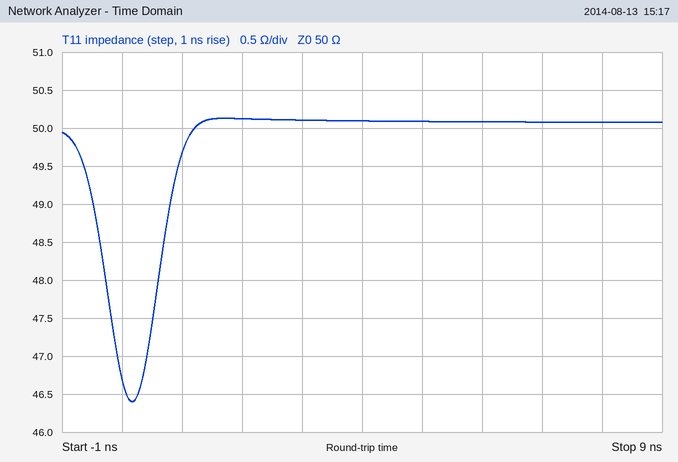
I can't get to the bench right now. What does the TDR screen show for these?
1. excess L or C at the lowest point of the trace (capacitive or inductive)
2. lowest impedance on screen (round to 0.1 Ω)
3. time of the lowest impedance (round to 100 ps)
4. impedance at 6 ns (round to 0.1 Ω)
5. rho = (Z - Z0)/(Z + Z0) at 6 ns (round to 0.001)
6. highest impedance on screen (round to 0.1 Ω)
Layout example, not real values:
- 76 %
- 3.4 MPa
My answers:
- capacitive
- 46.4 Ω
- 200 ps
- 50.1 Ω
- +0.001
- 50.1 Ω
